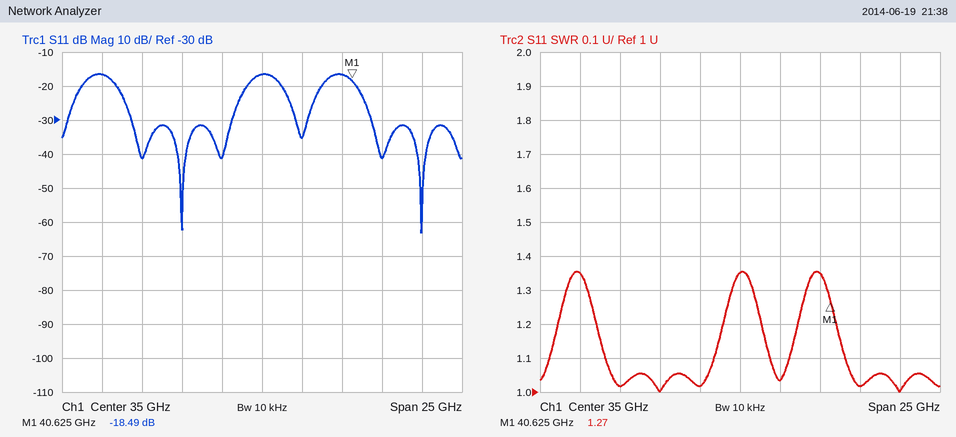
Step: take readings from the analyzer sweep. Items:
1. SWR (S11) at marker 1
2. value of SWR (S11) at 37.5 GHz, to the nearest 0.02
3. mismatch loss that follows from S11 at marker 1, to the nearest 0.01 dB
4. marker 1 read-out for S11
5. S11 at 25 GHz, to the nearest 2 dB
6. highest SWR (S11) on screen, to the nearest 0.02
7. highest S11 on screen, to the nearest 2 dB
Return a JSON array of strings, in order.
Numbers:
["1.27", "1.04", "0.06 dB", "-18.49 dB", "-16 dB", "1.36", "-16 dB"]
